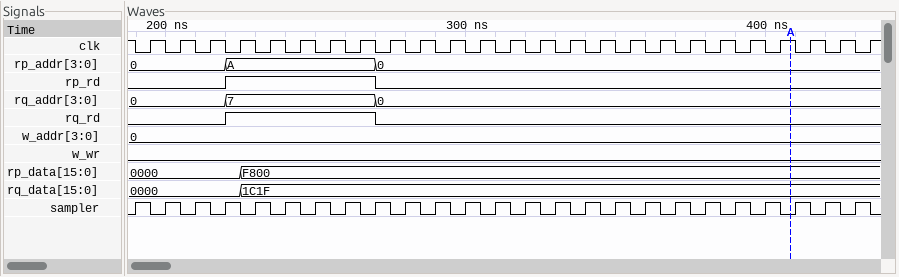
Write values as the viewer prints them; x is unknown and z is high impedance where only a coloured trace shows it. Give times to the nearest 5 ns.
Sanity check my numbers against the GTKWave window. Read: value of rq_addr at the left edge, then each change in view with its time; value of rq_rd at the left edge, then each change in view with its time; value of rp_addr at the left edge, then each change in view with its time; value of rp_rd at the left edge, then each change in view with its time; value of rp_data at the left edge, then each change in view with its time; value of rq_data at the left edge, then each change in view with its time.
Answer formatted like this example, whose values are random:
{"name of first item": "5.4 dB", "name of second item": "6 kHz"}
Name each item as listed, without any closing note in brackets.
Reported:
{"value of rq_addr at the left edge, then each change in view with its time": "0, 7 at 220 ns, 0 at 270 ns", "value of rq_rd at the left edge, then each change in view with its time": "0, 1 at 220 ns, 0 at 270 ns", "value of rp_addr at the left edge, then each change in view with its time": "0, A at 220 ns, 0 at 270 ns", "value of rp_rd at the left edge, then each change in view with its time": "0, 1 at 220 ns, 0 at 270 ns", "value of rp_data at the left edge, then each change in view with its time": "0000, F800 at 225 ns", "value of rq_data at the left edge, then each change in view with its time": "0000, 1C1F at 225 ns"}
